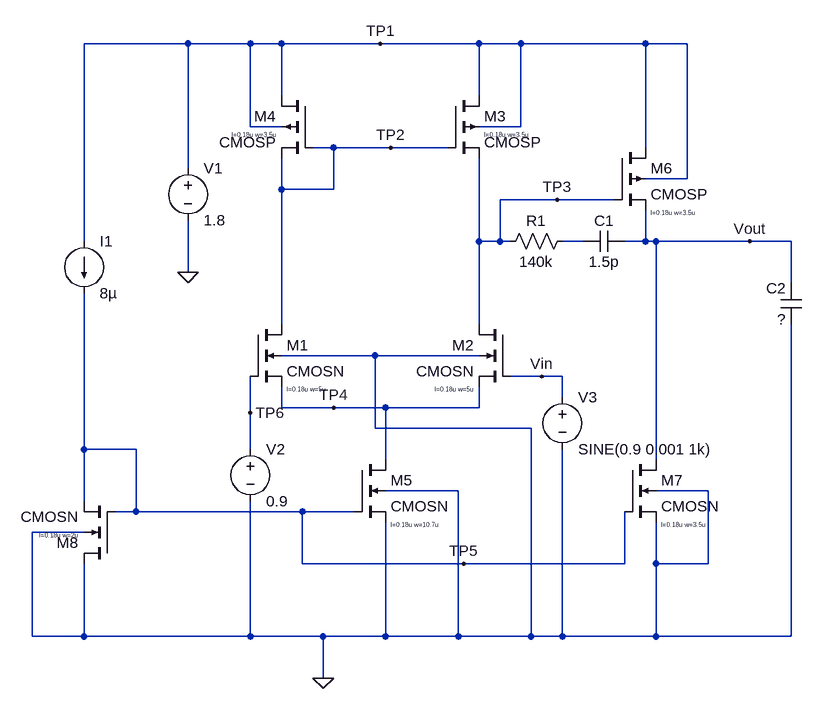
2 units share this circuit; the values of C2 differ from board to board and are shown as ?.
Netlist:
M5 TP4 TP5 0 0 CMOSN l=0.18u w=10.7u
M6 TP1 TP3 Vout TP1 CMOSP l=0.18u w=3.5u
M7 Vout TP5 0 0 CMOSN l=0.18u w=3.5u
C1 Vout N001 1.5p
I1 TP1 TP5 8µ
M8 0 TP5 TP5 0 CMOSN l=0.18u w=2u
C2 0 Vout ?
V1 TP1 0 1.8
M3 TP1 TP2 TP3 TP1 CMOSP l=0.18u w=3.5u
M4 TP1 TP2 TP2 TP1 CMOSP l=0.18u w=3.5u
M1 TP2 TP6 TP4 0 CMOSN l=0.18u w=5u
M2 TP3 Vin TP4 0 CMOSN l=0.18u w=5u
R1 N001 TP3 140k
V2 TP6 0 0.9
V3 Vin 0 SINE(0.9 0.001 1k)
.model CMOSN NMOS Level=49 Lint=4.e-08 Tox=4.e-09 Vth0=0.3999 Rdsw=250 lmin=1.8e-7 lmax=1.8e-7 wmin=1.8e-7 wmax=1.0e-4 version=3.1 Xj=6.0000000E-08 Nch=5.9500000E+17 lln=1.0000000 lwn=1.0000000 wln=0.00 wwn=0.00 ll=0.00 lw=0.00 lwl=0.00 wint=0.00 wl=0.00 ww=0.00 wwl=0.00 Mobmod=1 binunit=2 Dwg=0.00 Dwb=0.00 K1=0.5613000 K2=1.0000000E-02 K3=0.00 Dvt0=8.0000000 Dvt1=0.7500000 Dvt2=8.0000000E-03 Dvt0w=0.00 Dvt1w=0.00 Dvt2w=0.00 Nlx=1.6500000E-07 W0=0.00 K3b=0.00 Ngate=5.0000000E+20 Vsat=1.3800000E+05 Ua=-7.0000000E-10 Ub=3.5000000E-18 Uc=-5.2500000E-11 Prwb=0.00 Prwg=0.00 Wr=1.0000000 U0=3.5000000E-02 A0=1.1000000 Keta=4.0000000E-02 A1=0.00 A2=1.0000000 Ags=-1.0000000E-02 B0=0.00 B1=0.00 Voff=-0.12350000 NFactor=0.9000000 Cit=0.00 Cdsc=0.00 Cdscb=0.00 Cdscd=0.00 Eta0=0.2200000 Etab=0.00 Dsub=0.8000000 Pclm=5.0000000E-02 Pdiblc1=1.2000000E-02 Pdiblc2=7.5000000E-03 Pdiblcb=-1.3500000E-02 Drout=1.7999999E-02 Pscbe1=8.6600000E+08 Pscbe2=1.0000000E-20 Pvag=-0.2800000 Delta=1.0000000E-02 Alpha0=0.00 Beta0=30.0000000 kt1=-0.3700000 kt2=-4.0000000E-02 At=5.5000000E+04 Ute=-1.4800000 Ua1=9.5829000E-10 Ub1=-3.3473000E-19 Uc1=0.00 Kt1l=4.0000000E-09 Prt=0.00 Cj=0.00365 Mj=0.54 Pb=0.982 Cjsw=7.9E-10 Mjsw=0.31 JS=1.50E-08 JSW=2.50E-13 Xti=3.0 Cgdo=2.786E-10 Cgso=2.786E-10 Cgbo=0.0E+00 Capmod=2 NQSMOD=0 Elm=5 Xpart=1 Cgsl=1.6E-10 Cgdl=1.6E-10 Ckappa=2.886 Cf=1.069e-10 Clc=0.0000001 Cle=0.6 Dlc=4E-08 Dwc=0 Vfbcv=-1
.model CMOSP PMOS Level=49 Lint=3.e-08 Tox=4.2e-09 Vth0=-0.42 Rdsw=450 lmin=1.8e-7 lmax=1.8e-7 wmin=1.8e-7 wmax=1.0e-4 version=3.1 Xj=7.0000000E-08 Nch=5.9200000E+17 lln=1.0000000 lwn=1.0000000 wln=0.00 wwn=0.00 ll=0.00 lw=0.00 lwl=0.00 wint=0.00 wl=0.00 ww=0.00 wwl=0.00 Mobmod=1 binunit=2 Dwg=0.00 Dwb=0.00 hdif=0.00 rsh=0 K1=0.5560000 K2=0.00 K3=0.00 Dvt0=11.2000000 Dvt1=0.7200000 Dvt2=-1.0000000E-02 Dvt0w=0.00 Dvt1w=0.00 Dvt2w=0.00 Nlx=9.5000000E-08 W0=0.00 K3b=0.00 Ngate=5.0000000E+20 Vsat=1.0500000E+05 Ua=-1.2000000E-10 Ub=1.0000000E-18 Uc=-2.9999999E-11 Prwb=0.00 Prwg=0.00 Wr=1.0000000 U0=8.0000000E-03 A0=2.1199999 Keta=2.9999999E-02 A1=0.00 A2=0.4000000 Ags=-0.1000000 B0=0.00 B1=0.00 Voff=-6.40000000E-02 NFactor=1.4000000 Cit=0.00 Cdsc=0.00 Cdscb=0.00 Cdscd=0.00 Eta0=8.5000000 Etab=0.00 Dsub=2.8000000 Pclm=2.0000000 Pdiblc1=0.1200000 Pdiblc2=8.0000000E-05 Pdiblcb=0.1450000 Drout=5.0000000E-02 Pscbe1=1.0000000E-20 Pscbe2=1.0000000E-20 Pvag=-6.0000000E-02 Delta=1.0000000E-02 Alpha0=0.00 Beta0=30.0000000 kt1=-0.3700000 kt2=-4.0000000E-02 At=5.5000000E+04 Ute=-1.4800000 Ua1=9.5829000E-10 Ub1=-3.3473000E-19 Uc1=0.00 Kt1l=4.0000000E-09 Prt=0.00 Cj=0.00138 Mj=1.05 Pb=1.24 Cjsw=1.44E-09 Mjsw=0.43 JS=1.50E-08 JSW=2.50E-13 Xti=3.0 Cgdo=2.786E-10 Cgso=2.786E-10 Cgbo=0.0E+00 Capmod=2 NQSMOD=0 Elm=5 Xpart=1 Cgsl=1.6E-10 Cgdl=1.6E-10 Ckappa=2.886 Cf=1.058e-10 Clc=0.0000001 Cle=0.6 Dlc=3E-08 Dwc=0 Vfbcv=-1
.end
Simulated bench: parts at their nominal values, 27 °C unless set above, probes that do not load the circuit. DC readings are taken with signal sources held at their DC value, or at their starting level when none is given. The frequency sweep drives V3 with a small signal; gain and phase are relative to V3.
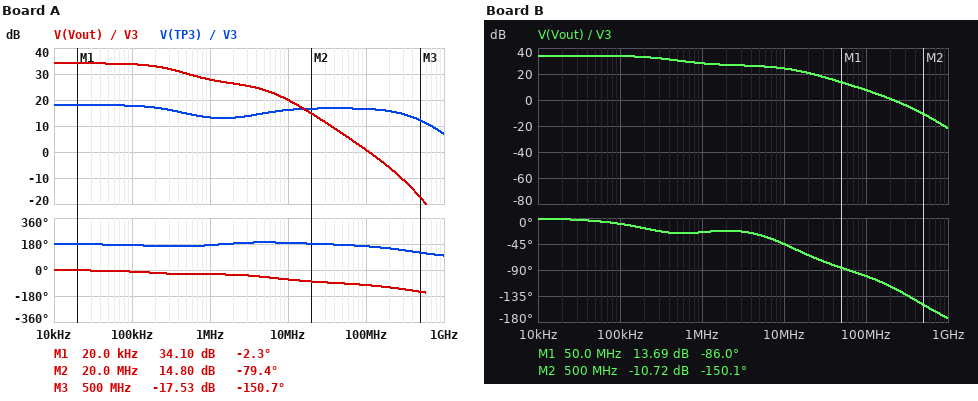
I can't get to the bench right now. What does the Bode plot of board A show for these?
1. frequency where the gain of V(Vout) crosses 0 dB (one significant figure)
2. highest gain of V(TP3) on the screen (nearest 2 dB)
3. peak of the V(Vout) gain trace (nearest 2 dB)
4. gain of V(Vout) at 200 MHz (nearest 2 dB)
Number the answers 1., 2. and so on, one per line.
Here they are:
1. 100 MHz
2. 18 dB
3. 34 dB
4. -6 dB
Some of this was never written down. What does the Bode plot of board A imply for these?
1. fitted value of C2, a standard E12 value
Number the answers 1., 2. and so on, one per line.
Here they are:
1. 3.3 pF
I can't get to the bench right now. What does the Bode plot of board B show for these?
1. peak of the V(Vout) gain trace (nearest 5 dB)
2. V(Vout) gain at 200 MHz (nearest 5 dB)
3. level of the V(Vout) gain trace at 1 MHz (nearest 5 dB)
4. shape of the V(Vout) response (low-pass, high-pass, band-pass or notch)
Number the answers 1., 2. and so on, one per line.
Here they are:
1. 35 dB
2. 0 dB
3. 30 dB
4. low-pass
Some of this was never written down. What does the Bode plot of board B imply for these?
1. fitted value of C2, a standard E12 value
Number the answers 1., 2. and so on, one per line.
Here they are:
1. 1.5 pF
